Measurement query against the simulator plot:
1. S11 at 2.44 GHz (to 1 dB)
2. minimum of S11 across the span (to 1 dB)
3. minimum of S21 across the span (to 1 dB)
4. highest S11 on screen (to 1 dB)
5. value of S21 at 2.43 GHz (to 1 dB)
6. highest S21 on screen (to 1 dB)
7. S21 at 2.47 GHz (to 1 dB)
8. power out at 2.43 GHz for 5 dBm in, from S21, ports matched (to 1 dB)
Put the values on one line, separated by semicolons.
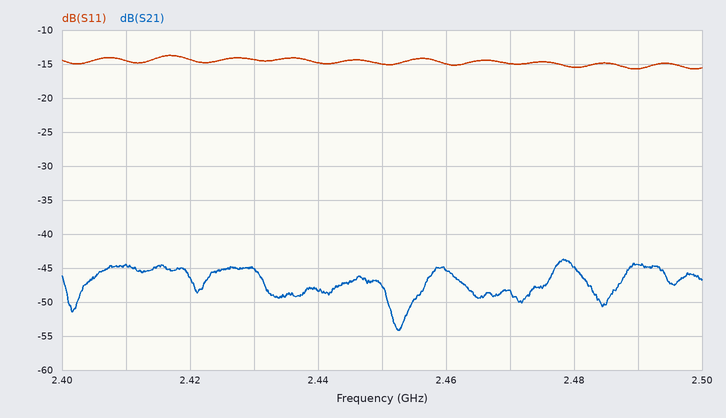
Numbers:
-15 dB; -16 dB; -54 dB; -14 dB; -45 dB; -44 dB; -48 dB; -40 dBm
